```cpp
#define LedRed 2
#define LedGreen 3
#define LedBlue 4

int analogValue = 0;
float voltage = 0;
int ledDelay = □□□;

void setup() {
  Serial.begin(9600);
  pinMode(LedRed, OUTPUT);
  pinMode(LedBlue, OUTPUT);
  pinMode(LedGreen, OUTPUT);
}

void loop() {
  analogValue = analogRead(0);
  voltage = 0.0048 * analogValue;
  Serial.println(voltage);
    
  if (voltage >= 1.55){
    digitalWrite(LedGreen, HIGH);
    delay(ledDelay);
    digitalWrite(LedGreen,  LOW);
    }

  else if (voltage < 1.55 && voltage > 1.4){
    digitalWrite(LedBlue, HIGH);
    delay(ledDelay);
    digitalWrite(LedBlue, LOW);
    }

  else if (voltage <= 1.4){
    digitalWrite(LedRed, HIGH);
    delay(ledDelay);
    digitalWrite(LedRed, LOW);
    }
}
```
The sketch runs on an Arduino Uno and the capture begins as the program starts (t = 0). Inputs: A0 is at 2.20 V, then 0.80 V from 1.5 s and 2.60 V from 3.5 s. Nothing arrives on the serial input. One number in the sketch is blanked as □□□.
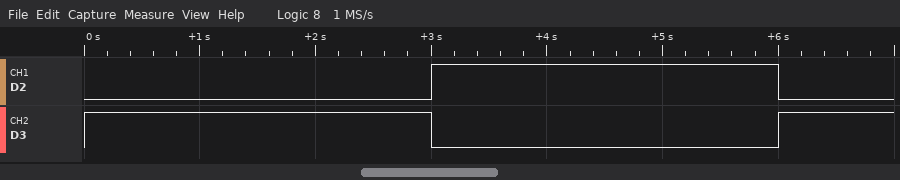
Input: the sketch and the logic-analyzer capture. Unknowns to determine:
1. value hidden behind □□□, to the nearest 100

3000
